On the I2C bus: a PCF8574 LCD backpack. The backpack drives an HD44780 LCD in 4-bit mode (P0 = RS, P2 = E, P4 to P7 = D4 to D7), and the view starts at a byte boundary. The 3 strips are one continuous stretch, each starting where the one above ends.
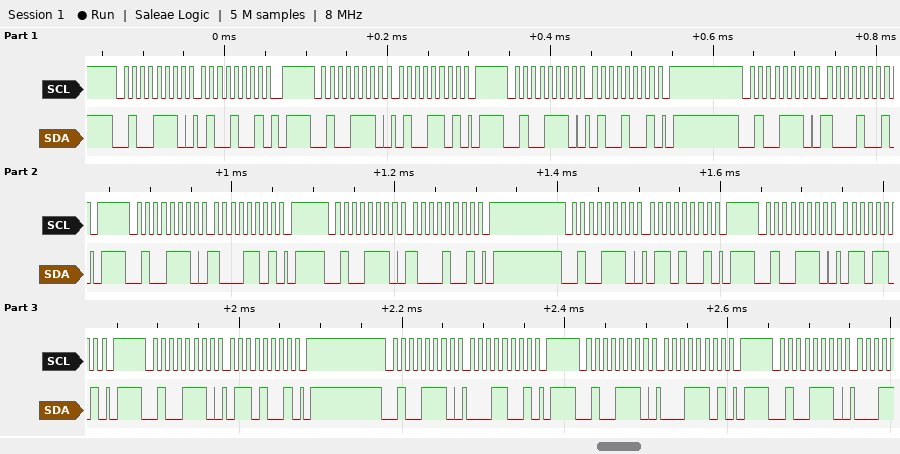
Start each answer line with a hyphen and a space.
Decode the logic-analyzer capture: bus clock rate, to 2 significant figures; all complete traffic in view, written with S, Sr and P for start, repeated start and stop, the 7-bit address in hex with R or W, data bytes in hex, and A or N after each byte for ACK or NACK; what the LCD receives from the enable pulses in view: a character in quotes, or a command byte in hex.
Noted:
- 100 kHz
- S 27W A 49 A P S 27W A 4D A P S 27W A 49 A P S 27W A 89 A P S 27W A 8D A P S 27W A 89 A P S 27W A 69 A P S 27W A 6D A P S 27W A 69 A P S 27W A 19 A P S 27W A 1D A P S 27W A
- 'H'
